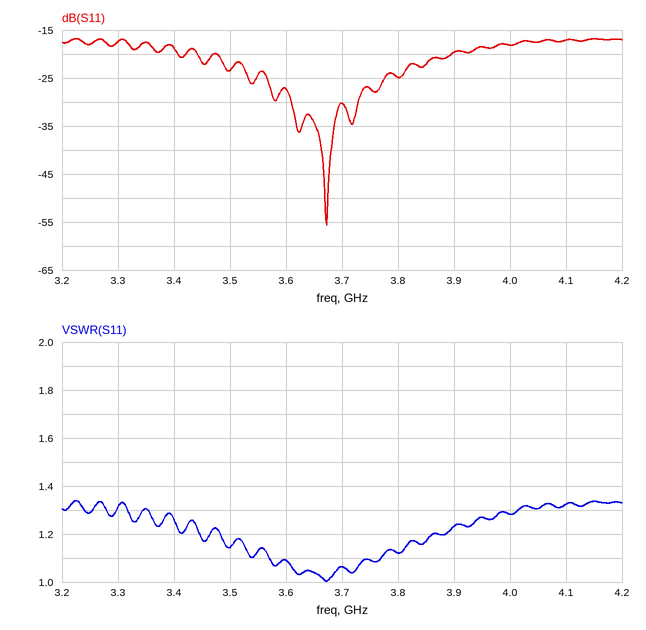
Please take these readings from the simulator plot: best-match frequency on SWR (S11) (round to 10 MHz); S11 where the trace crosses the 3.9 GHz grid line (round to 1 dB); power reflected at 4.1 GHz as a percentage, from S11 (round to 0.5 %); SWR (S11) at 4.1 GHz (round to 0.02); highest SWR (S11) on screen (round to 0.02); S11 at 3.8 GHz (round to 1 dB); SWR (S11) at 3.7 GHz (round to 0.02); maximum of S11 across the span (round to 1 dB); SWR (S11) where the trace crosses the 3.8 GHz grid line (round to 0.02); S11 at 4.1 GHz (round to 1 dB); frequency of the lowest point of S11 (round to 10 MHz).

3.67 GHz
-20 dB
2.0 %
1.32
1.34
-25 dB
1.06
-17 dB
1.12
-17 dB
3.67 GHz
